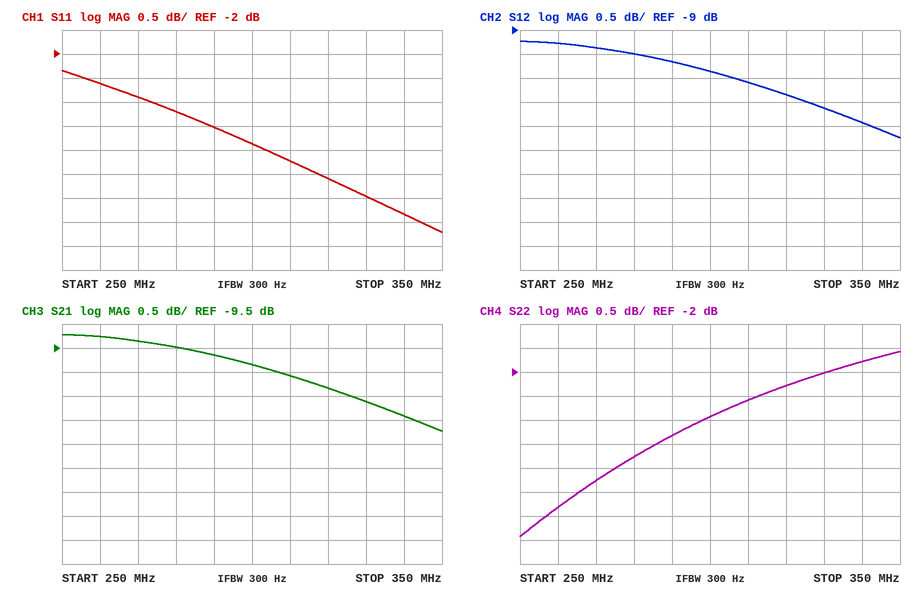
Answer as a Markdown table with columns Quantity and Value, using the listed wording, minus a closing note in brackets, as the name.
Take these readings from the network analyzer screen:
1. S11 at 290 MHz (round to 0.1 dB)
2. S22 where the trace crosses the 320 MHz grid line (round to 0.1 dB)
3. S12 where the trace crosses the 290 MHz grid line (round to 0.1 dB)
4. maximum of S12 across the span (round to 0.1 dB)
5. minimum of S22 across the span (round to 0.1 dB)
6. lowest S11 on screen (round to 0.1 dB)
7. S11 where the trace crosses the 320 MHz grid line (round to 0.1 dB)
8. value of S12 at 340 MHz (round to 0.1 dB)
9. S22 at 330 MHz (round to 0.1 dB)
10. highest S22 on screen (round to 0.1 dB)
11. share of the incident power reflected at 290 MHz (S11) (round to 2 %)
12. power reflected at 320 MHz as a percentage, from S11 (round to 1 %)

| Quantity | Value |
|---|---|
| S11 at 290 MHz | -3.5 dB |
| S22 where the trace crosses the 320 MHz grid line | -2.3 dB |
| S12 where the trace crosses the 290 MHz grid line | -9.7 dB |
| maximum of S12 across the span | -9.2 dB |
| minimum of S22 across the span | -5.4 dB |
| lowest S11 on screen | -5.7 dB |
| S11 where the trace crosses the 320 MHz grid line | -4.6 dB |
| value of S12 at 340 MHz | -10.9 dB |
| S22 at 330 MHz | -2.0 dB |
| highest S22 on screen | -1.6 dB |
| share of the incident power reflected at 290 MHz (S11) | 44 % |
| power reflected at 320 MHz as a percentage, from S11 | 35 % |
